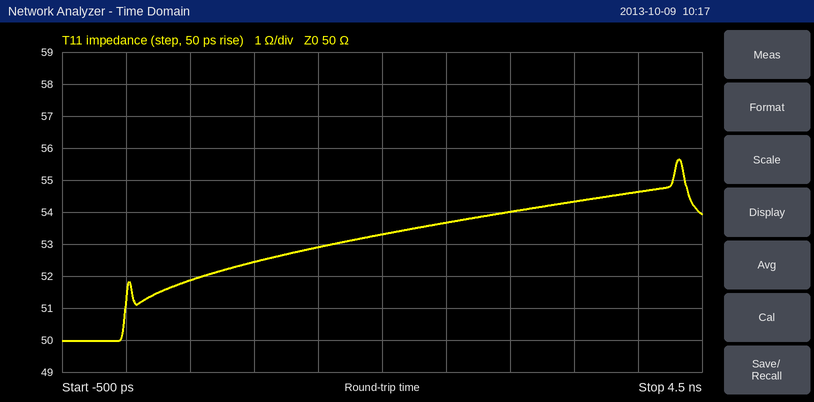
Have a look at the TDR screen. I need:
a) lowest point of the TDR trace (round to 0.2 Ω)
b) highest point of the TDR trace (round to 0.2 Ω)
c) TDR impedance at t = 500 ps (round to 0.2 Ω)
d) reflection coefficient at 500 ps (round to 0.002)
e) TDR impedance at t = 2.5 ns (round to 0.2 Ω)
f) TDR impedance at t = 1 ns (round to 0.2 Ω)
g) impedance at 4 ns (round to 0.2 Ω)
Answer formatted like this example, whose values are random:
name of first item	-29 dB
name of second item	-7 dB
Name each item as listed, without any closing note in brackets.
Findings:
lowest point of the TDR trace	50.0 Ω
highest point of the TDR trace	55.6 Ω
TDR impedance at t = 500 ps	51.8 Ω
reflection coefficient at 500 ps	+0.018
TDR impedance at t = 2.5 ns	53.6 Ω
TDR impedance at t = 1 ns	52.4 Ω
impedance at 4 ns	54.6 Ω
